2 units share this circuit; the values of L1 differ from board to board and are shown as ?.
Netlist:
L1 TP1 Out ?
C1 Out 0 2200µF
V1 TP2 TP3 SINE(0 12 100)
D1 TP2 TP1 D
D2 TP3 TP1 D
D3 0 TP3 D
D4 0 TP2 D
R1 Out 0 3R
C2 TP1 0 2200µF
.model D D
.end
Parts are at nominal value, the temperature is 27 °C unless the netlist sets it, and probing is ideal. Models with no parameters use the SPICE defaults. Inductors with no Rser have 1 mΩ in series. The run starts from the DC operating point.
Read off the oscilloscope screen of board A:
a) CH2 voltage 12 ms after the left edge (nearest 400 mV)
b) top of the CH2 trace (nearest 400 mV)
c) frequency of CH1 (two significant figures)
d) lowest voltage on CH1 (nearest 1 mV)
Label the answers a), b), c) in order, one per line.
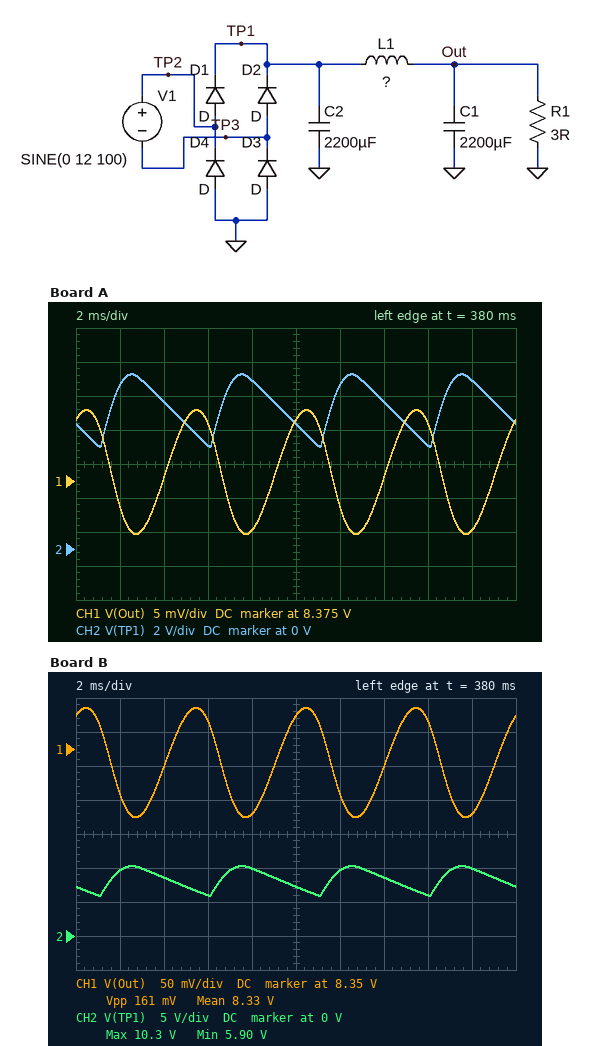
a) 9.6 V
b) 10.4 V
c) 200 Hz
d) 8.367 V
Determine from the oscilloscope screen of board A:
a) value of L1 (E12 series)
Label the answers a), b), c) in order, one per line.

a) 56 mH
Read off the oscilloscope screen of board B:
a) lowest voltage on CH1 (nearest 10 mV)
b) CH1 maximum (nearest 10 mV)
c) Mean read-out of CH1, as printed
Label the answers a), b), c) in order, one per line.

a) 8.25 V
b) 8.41 V
c) 8.33 V
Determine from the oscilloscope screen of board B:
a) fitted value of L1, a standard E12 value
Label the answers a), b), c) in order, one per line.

a) 6.8 mH
